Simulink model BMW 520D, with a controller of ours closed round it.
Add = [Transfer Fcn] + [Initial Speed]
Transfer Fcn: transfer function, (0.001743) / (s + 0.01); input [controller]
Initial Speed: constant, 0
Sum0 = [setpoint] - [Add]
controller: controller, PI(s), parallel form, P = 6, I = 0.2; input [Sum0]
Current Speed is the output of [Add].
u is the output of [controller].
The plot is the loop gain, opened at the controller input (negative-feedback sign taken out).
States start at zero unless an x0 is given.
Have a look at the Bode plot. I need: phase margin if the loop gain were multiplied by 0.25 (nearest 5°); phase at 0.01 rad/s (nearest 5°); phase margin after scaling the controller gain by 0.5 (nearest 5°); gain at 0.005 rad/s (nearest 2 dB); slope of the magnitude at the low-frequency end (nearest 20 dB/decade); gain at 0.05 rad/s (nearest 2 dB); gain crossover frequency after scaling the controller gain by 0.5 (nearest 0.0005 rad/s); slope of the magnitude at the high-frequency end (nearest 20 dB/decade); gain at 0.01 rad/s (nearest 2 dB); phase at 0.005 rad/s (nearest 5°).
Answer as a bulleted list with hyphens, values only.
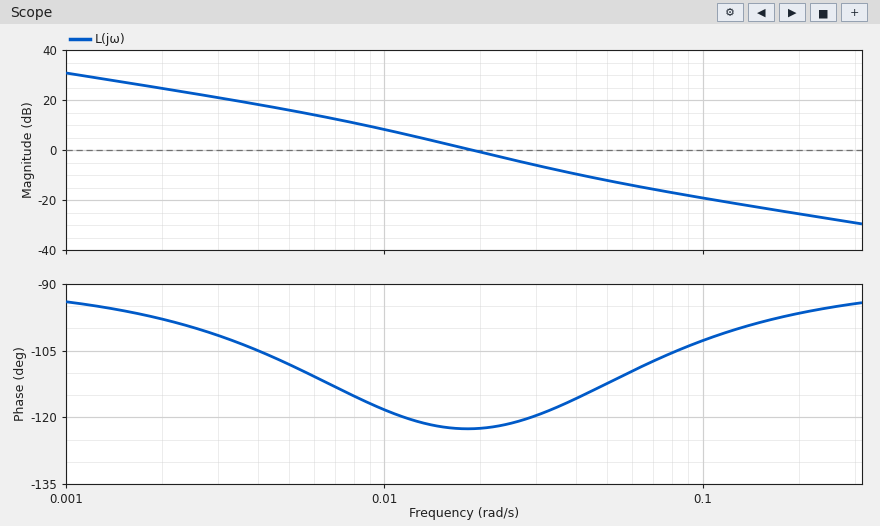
- 65°
- -120°
- 60°
- 16 dB
- -20 dB/decade
- -12 dB
- 0.0120 rad/s
- -20 dB/decade
- 8 dB
- -110°
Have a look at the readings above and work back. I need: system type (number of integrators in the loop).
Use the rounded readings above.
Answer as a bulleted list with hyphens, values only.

- 1
